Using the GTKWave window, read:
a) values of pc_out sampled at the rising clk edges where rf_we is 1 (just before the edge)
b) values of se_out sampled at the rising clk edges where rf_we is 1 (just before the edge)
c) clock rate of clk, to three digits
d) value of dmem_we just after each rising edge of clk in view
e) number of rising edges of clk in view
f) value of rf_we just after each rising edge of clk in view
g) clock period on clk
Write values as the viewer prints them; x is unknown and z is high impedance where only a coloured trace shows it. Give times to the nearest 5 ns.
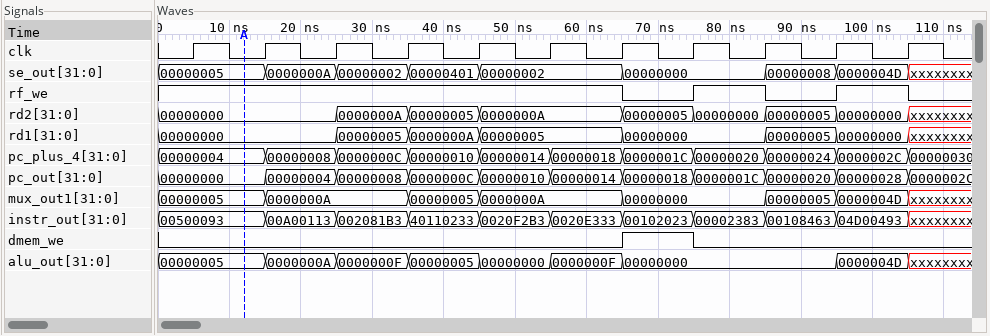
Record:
00000000, 00000000, 00000004, 00000008, 0000000C, 00000010, 00000014, 0000001C, 00000028
00000005, 00000005, 0000000A, 00000002, 00000401, 00000002, 00000002, 00000000, 0000004D
100 MHz
0 0 0 0 0 0 1 0 0 0 0
11
1 1 1 1 1 1 0 1 0 1 0
10 ns
